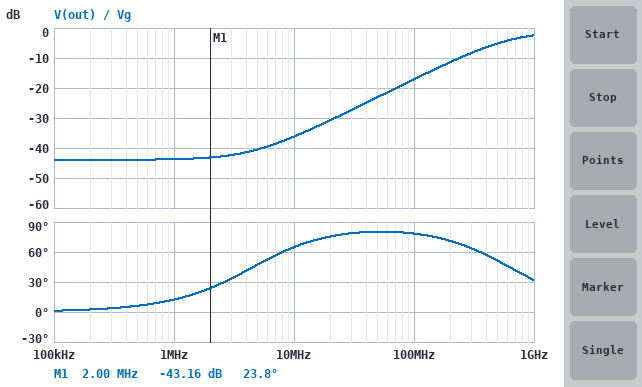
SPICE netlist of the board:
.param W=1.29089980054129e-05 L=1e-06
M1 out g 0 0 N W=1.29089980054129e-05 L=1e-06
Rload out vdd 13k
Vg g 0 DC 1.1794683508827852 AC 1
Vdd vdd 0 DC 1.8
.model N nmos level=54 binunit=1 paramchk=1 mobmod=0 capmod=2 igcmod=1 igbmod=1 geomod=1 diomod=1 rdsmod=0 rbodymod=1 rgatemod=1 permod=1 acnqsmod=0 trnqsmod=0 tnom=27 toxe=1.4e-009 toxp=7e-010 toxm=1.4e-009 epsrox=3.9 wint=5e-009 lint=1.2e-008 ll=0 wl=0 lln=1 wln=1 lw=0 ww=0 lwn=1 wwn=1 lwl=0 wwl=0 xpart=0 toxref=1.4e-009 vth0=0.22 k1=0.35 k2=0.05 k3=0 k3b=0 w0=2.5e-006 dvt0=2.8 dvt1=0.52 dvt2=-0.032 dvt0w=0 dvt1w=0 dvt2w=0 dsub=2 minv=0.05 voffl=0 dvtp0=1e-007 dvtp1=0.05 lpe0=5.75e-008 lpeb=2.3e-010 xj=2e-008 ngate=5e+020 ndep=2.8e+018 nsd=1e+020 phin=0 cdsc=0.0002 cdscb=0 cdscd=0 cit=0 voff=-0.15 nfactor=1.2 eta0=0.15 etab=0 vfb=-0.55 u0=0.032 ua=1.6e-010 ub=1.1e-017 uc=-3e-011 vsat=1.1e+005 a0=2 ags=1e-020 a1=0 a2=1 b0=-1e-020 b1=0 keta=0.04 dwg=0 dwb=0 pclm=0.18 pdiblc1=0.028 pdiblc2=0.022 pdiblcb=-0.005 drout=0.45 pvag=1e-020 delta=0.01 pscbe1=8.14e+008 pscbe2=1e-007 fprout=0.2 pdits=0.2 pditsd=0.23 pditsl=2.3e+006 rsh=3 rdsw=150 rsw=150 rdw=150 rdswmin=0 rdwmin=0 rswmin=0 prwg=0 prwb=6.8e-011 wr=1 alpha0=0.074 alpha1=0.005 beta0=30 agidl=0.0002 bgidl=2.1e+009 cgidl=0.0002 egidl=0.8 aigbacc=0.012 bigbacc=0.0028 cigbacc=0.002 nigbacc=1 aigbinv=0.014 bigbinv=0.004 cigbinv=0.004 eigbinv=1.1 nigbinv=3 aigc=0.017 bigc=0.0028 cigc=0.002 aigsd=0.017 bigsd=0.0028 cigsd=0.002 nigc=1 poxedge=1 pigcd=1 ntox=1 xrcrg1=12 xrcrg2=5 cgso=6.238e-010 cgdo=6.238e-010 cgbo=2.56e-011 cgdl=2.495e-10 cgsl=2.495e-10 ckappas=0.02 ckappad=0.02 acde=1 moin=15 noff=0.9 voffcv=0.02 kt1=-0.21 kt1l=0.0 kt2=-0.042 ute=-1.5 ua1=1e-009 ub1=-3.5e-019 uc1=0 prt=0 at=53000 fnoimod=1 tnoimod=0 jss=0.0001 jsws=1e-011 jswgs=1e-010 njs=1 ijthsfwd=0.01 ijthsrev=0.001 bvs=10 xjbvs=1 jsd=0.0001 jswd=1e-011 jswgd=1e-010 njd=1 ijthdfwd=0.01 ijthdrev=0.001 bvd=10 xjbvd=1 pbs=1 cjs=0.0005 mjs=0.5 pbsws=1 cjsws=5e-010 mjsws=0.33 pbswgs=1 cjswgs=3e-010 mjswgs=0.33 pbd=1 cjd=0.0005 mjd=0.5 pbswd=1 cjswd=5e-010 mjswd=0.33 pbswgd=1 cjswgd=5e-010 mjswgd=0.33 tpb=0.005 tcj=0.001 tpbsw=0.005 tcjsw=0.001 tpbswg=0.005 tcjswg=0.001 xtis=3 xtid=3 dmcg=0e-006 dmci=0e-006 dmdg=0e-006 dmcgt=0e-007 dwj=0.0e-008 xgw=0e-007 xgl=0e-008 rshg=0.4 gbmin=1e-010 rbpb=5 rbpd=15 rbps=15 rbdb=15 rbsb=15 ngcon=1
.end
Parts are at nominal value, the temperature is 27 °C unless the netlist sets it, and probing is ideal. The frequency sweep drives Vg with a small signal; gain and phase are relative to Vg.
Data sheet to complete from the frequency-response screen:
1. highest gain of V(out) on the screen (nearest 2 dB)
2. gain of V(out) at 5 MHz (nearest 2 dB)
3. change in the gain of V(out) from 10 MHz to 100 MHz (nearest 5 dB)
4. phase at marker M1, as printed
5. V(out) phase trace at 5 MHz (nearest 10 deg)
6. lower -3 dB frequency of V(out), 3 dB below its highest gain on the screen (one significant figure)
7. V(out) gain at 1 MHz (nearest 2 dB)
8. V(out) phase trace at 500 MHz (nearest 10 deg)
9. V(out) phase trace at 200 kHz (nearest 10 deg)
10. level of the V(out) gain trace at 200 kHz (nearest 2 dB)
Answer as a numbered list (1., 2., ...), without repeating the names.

1. -2 dB
2. -40 dB
3. 20 dB
4. 23.8 deg
5. 50 deg
6. 500 MHz
7. -44 dB
8. 50 deg
9. 0 deg
10. -44 dB
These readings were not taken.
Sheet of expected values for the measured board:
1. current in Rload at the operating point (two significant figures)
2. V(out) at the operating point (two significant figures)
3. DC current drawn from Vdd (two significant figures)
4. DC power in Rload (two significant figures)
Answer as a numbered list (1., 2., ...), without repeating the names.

1. 130 µA
2. 110 mV
3. 130 µA
4. 220 µW
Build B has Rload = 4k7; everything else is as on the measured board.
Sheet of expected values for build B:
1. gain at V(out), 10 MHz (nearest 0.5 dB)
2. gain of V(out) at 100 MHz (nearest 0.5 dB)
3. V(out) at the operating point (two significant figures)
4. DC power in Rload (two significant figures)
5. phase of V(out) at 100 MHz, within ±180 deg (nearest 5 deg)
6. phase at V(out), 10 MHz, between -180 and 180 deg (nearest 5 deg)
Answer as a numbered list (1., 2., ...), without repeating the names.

1. -23.0 dB
2. -15.5 dB
3. 320 mV
4. 470 µW
5. 105 deg
6. 165 deg
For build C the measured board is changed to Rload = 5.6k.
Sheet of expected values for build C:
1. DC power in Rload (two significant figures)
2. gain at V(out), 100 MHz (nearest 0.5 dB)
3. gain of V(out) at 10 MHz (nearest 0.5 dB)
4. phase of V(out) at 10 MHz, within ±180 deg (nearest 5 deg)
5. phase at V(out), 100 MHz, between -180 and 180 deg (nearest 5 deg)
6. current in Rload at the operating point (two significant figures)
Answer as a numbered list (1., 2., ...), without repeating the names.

1. 420 µW
2. -16.0 dB
3. -28.0 dB
4. 155 deg
5. 95 deg
6. 270 µA
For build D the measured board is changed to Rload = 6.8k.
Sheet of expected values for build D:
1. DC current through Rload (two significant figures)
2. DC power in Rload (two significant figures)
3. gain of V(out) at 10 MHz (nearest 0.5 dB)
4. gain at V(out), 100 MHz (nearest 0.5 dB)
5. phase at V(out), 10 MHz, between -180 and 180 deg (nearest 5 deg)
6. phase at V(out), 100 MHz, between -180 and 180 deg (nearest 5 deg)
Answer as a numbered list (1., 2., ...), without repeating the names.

1. 230 µA
2. 370 µW
3. -33.5 dB
4. -16.5 dB
5. 135 deg
6. 85 deg
